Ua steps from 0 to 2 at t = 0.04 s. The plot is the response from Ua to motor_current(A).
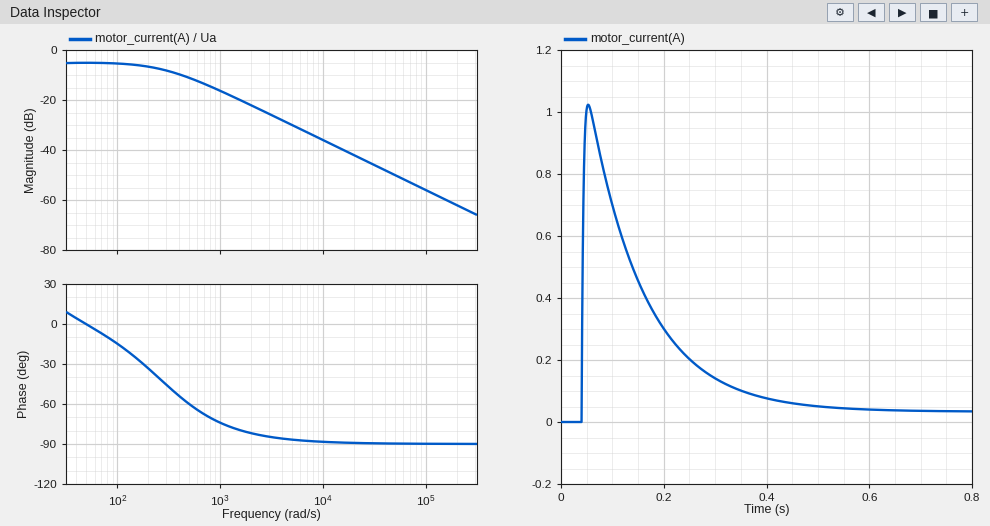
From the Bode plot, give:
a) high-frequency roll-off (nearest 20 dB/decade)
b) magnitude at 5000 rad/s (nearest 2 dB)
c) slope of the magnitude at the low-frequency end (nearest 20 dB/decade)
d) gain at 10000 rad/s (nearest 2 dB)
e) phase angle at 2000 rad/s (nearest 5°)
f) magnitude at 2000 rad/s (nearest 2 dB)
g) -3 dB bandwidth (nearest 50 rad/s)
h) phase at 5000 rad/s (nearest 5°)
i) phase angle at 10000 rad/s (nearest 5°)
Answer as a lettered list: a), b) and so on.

a) -20 dB/decade
b) -30 dB
c) 0 dB/decade
d) -36 dB
e) -80°
f) -22 dB
g) 300 rad/s
h) -85°
i) -90°
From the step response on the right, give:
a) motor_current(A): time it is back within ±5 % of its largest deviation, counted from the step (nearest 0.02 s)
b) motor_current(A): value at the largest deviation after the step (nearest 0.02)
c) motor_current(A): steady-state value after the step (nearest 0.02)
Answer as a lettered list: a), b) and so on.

a) 0.34 s
b) 1.02
c) 0.04
